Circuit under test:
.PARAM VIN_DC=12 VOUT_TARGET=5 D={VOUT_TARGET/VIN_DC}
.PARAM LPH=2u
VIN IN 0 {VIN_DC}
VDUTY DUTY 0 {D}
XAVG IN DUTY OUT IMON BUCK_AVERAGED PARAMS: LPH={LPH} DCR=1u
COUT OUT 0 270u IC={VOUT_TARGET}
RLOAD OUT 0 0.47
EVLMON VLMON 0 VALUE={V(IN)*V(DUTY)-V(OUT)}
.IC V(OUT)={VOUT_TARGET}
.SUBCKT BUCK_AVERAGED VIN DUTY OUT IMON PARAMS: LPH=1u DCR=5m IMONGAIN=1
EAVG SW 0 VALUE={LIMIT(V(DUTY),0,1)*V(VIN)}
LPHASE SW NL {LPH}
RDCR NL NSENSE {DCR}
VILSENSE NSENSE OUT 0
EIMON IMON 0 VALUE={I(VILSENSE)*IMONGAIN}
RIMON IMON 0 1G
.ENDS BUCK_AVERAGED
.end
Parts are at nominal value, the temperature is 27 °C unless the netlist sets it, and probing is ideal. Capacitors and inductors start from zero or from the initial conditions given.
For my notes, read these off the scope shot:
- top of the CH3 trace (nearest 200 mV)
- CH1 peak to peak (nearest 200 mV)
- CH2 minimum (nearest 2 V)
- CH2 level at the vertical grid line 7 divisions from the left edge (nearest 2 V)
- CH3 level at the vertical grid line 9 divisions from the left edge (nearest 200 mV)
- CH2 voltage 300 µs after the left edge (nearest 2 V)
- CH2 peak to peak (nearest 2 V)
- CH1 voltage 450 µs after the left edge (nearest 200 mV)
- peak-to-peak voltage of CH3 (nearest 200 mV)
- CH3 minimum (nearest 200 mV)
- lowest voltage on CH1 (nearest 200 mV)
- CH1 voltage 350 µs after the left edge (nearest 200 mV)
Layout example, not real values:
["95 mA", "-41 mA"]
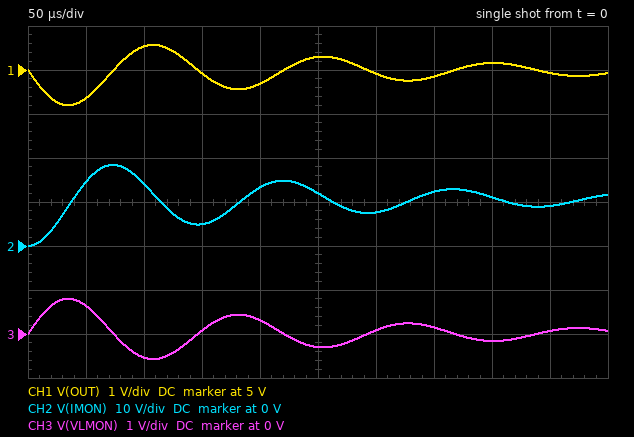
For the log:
["800 mV", "1.4 V", "0 V", "12 V", "0 V", "8 V", "18 V", "5.0 V", "1.4 V", "-600 mV", "4.2 V", "4.8 V"]
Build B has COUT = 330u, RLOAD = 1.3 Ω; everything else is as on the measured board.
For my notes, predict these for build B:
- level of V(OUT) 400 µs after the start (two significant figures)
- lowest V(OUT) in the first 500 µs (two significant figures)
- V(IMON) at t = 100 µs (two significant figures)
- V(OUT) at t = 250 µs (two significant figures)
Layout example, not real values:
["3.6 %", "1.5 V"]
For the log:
["5.0 V", "4.7 V", "6.4 V", "5.1 V"]
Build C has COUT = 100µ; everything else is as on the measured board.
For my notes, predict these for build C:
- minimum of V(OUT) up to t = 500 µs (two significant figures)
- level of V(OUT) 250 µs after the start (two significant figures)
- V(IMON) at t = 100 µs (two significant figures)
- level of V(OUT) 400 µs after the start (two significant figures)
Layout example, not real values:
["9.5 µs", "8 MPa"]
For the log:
["3.8 V", "5.1 V", "7.5 V", "5.0 V"]
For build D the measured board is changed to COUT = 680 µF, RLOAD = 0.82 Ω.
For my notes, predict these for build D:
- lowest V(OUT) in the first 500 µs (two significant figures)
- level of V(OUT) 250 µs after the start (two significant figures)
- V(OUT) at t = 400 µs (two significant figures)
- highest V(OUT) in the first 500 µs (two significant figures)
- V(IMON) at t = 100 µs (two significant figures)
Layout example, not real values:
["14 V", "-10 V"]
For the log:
["4.7 V", "4.9 V", "5.2 V", "5.3 V", "11 V"]
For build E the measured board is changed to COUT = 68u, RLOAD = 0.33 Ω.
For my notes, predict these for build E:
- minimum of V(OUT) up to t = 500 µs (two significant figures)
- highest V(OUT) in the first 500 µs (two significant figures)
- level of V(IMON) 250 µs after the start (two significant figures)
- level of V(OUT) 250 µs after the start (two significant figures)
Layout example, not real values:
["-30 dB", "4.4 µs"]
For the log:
["3.2 V", "5.8 V", "15 V", "5.0 V"]
